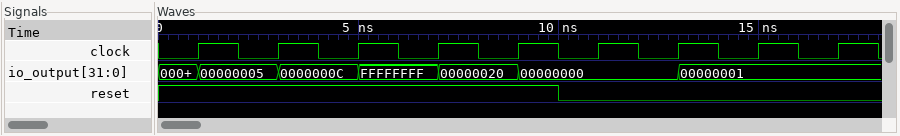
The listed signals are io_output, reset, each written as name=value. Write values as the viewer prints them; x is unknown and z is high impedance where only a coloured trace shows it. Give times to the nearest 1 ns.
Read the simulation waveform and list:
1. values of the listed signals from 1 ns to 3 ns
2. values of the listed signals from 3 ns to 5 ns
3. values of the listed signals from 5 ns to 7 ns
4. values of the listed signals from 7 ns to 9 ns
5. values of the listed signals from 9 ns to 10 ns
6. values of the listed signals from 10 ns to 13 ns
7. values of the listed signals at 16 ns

io_output=00000005, reset=1
io_output=0000000C, reset=1
io_output=FFFFFFFF, reset=1
io_output=00000020, reset=1
io_output=00000000, reset=1
io_output=00000000, reset=0
io_output=00000001, reset=0
